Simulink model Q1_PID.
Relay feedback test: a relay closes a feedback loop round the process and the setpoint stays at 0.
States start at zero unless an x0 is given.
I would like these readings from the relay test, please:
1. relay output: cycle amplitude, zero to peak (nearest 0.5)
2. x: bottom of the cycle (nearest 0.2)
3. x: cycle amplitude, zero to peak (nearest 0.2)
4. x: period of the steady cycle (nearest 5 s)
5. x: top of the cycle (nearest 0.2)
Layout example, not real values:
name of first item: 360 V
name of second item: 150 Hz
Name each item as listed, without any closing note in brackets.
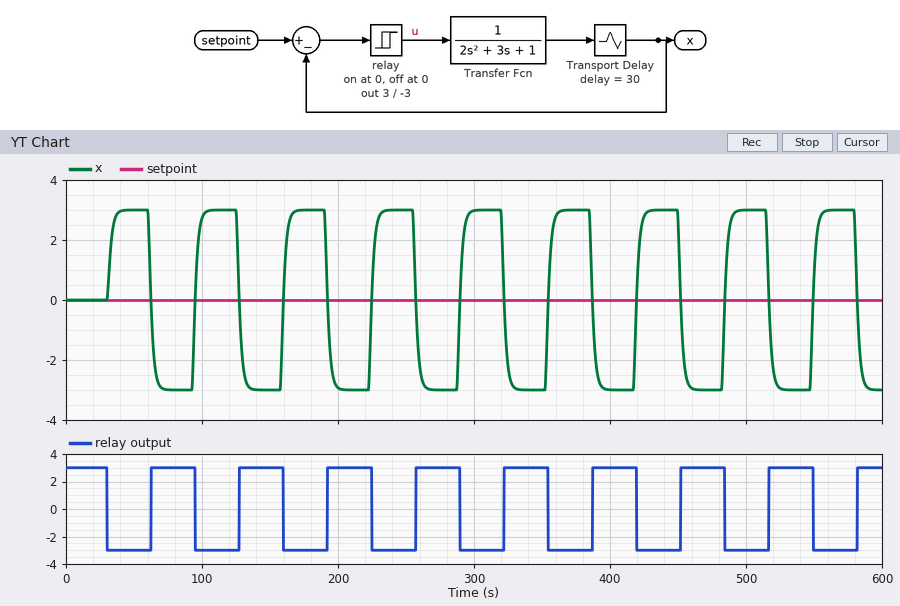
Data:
relay output: cycle amplitude, zero to peak: 3.0
x: bottom of the cycle: -3.0
x: cycle amplitude, zero to peak: 3.0
x: period of the steady cycle: 65 s
x: top of the cycle: 3.0
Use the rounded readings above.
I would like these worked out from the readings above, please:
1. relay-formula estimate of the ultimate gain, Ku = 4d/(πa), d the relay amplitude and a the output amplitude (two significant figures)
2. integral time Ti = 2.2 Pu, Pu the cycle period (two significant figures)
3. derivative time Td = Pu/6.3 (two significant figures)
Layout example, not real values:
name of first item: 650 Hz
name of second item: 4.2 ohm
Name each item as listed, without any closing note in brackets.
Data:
relay-formula estimate of the ultimate gain, Ku = 4d/(πa), d the relay amplitude and a the output amplitude: 1.3
integral time Ti = 2.2 Pu, Pu the cycle period: 140 s
derivative time Td = Pu/6.3: 10 s
